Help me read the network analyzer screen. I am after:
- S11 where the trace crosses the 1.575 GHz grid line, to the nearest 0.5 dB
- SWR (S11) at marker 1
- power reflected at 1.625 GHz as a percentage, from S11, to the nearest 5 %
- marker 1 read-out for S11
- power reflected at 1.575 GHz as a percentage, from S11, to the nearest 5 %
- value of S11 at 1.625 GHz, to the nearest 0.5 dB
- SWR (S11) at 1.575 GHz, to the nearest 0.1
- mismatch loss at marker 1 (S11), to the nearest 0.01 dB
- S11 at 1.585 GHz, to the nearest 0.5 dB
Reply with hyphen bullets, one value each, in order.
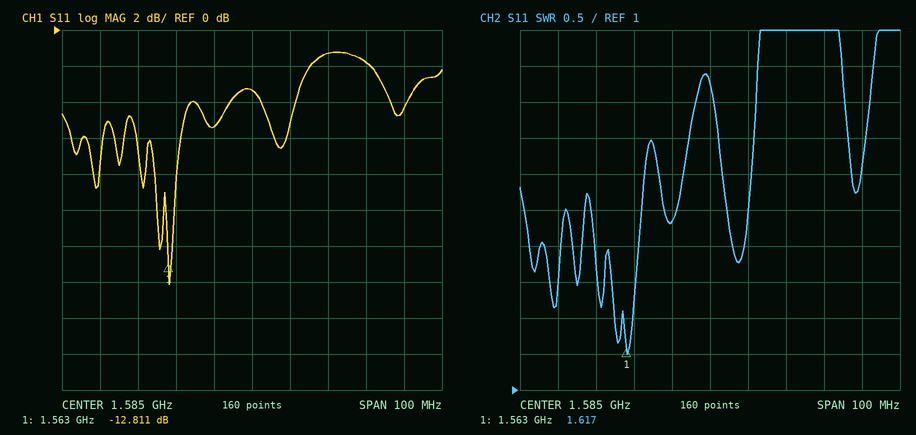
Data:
- -5.5 dB
- 1.617
- 35 %
- -12.811 dB
- 30 %
- -4.5 dB
- 3.3
- 0.23 dB
- -3.5 dB
